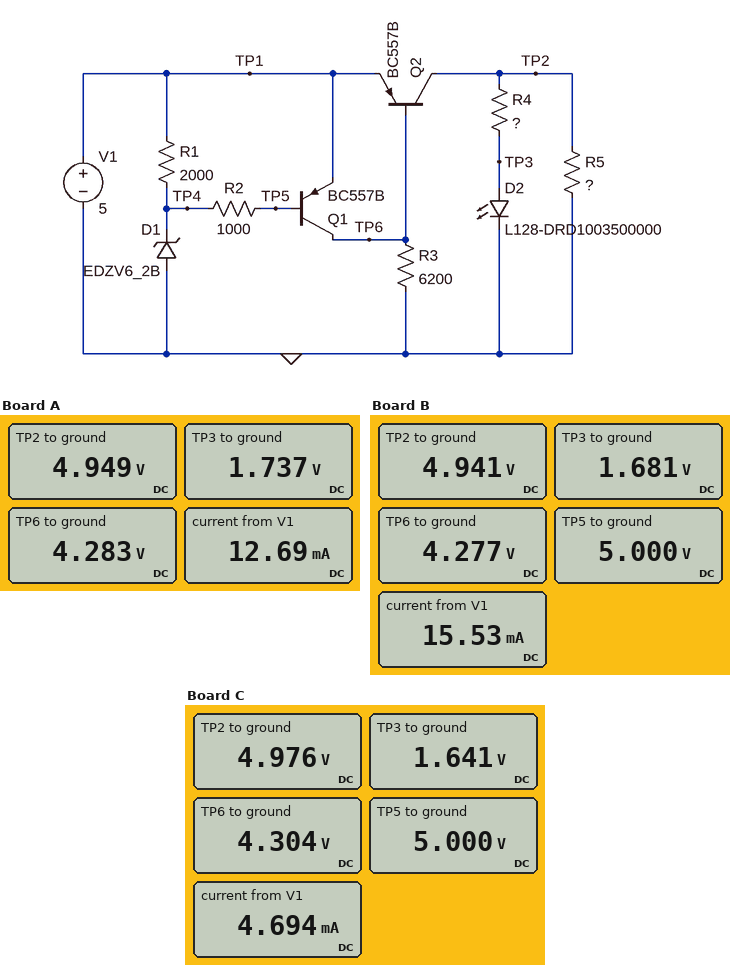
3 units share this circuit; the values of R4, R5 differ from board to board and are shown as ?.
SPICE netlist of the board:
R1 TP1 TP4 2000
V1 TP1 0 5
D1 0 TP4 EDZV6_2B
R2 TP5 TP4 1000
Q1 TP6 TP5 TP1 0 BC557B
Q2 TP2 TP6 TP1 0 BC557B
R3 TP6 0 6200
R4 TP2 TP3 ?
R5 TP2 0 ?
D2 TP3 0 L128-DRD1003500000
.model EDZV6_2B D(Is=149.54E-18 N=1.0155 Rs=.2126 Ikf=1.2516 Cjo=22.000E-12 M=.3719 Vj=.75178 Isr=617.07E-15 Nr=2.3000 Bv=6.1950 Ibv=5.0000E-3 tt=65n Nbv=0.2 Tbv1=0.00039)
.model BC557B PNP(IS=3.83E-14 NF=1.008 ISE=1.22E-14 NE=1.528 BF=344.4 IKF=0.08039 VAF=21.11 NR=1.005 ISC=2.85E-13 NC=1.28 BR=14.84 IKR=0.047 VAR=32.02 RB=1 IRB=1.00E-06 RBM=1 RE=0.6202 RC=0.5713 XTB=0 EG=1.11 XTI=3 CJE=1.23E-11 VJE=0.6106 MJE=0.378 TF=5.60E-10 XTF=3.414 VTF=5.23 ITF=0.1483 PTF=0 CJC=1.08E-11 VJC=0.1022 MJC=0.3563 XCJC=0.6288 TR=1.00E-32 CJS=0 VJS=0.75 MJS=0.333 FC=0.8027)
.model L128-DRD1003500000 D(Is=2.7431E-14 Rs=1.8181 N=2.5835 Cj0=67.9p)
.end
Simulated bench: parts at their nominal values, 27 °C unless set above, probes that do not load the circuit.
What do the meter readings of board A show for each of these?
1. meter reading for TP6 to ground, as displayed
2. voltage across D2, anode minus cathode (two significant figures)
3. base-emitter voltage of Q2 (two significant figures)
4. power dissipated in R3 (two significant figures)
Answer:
4.283 V
1.7 V
-720 mV
3.0 mW
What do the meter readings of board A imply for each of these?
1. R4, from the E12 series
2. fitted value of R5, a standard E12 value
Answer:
680 Ω
680 Ω
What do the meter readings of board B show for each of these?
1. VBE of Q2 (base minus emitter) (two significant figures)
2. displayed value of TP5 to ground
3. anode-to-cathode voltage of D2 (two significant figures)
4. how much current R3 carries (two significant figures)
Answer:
-720 mV
5.000 V
1.7 V
690 µA
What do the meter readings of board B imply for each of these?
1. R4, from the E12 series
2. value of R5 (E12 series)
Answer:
1.5 kΩ
390 Ω
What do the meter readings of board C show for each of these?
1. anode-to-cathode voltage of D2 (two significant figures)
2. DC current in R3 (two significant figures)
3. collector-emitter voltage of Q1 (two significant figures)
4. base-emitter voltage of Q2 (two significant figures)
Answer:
1.6 V
690 µA
-700 mV
-700 mV
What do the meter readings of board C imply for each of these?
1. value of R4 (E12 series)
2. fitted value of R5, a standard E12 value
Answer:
2.7 kΩ
1.8 kΩ
